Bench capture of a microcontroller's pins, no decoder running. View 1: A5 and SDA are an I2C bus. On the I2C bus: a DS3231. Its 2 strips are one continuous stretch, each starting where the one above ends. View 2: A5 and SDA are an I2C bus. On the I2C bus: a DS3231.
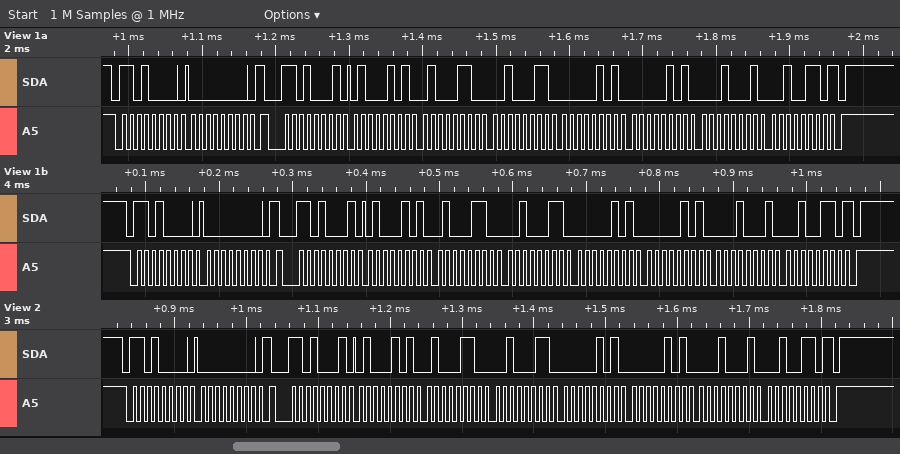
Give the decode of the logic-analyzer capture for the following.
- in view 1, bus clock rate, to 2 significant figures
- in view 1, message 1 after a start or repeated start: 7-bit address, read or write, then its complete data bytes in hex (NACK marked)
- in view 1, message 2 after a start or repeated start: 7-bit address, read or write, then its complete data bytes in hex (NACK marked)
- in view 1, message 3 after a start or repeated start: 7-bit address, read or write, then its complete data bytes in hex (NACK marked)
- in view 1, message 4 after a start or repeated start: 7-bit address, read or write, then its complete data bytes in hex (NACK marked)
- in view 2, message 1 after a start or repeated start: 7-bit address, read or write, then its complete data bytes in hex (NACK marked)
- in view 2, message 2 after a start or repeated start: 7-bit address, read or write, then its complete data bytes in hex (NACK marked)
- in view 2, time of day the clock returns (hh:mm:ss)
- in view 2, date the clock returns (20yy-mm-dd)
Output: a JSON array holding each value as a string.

["100 kHz", "0x68 write: 00", "0x68 read: 45 46 23 05 05 11 26 NACK", "0x68 write: 00", "0x68 read: 45 46 23 05 05 11 26 NACK", "0x68 write: 00", "0x68 read: 45 46 23 05 05 11 26 NACK", "23:46:45", "2026-11-05"]
